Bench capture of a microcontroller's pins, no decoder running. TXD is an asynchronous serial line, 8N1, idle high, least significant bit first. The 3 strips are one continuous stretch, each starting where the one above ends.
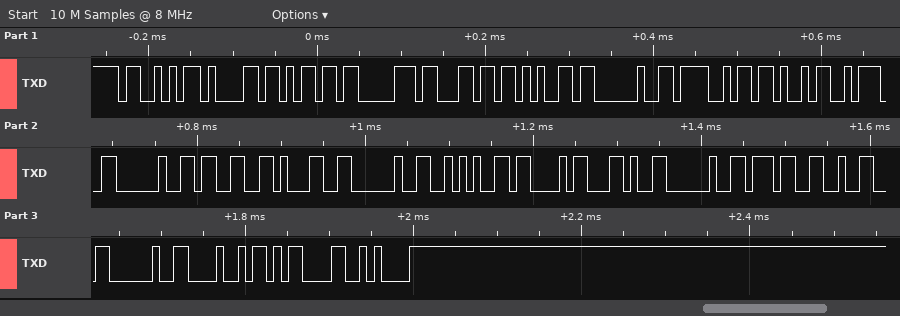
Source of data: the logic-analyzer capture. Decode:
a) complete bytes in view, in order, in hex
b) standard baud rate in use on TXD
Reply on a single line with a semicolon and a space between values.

53 61 6D 70 6C 65 20 4F 4B 3A 20 33 31 20 2A 43 2C 20 37 32 20 48 0D 0A; 115200 baud
